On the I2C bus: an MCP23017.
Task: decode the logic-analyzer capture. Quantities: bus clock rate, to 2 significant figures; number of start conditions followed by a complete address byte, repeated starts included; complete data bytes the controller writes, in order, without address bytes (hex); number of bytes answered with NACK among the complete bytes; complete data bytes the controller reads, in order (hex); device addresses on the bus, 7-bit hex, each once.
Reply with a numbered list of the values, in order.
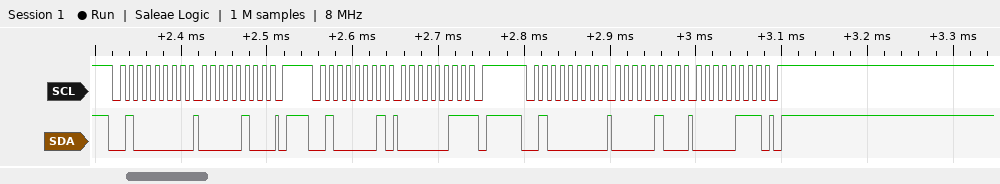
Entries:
1. 100 kHz
2. 3
3. 04 04 07
4. 1
5. 03
6. 0x20
